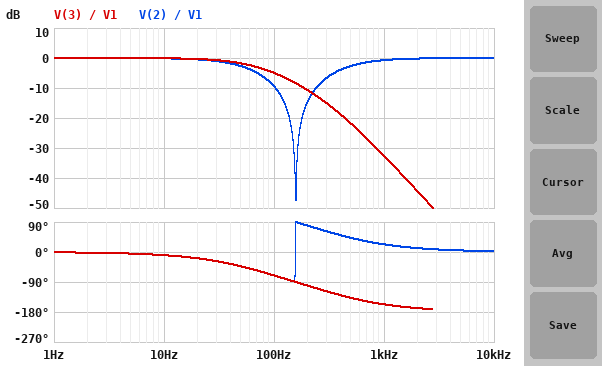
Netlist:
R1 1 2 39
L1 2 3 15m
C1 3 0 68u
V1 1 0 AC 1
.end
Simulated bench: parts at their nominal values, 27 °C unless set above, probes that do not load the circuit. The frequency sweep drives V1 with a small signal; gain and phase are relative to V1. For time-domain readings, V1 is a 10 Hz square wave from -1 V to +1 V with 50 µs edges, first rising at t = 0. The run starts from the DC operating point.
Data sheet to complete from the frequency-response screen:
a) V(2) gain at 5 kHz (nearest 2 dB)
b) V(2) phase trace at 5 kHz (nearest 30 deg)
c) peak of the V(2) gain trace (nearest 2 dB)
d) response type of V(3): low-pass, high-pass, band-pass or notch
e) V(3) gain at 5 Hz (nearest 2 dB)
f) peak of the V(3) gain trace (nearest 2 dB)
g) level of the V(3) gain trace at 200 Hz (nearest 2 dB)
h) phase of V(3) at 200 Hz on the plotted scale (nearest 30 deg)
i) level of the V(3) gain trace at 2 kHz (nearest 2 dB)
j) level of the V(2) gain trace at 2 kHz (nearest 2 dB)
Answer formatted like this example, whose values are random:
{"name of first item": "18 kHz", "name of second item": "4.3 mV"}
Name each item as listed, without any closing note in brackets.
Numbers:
{"V(2) gain at 5 kHz": "0 dB", "V(2) phase trace at 5 kHz": "0 deg", "peak of the V(2) gain trace": "0 dB", "response type of V(3): low-pass, high-pass, band-pass or notch": "low-pass", "V(3) gain at 5 Hz": "0 dB", "peak of the V(3) gain trace": "0 dB", "level of the V(3) gain trace at 200 Hz": "-10 dB", "phase of V(3) at 200 Hz on the plotted scale": "-90 deg", "level of the V(3) gain trace at 2 kHz": "-44 dB", "level of the V(2) gain trace at 2 kHz": "0 dB"}
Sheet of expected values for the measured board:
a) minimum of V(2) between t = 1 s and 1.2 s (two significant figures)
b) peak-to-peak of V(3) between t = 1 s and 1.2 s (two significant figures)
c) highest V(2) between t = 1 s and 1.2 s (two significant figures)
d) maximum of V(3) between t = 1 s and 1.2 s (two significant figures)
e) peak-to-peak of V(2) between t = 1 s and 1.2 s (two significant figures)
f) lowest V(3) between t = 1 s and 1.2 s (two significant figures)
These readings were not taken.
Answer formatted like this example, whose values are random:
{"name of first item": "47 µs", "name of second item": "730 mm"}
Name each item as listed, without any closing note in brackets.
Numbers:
{"minimum of V(2) between t = 1 s and 1.2 s": "-1.0 V", "peak-to-peak of V(3) between t = 1 s and 1.2 s": "2.0 V", "highest V(2) between t = 1 s and 1.2 s": "1.0 V", "maximum of V(3) between t = 1 s and 1.2 s": "1.0 V", "peak-to-peak of V(2) between t = 1 s and 1.2 s": "2.0 V", "lowest V(3) between t = 1 s and 1.2 s": "-1.0 V"}
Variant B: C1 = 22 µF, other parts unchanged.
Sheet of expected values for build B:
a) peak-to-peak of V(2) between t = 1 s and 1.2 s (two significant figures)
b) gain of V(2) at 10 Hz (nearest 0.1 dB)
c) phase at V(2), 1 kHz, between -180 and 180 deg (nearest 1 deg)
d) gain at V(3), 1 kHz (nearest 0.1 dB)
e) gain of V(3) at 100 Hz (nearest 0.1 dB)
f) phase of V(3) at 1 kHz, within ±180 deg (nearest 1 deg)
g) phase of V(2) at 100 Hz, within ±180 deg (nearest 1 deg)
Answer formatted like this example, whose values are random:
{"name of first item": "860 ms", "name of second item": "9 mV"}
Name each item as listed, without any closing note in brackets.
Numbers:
{"peak-to-peak of V(2) between t = 1 s and 1.2 s": "2.1 V", "gain of V(2) at 10 Hz": "0 dB", "phase at V(2), 1 kHz, between -180 and 180 deg": "24 deg", "gain at V(3), 1 kHz": "-22.4 dB", "gain of V(3) at 100 Hz": "-0.2 dB", "phase of V(3) at 1 kHz, within ±180 deg": "-156 deg", "phase of V(2) at 100 Hz, within ±180 deg": "-32 deg"}
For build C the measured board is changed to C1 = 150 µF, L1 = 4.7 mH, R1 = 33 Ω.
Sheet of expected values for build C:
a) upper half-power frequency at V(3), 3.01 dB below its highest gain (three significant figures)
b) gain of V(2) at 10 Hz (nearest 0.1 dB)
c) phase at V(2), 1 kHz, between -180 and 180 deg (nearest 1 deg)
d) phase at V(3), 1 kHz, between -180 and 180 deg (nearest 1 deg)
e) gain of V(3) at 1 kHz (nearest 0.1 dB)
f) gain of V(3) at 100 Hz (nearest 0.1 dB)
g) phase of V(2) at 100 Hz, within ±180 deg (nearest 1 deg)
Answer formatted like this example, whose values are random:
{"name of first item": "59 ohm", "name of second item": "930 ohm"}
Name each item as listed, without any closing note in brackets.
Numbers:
{"upper half-power frequency at V(3), 3.01 dB below its highest gain": "33.1 Hz", "gain of V(2) at 10 Hz": "-0.4 dB", "phase at V(2), 1 kHz, between -180 and 180 deg": "49 deg", "phase at V(3), 1 kHz, between -180 and 180 deg": "-131 deg", "gain of V(3) at 1 kHz": "-32.3 dB", "gain of V(3) at 100 Hz": "-10.1 dB", "phase of V(2) at 100 Hz, within ±180 deg": "-77 deg"}
